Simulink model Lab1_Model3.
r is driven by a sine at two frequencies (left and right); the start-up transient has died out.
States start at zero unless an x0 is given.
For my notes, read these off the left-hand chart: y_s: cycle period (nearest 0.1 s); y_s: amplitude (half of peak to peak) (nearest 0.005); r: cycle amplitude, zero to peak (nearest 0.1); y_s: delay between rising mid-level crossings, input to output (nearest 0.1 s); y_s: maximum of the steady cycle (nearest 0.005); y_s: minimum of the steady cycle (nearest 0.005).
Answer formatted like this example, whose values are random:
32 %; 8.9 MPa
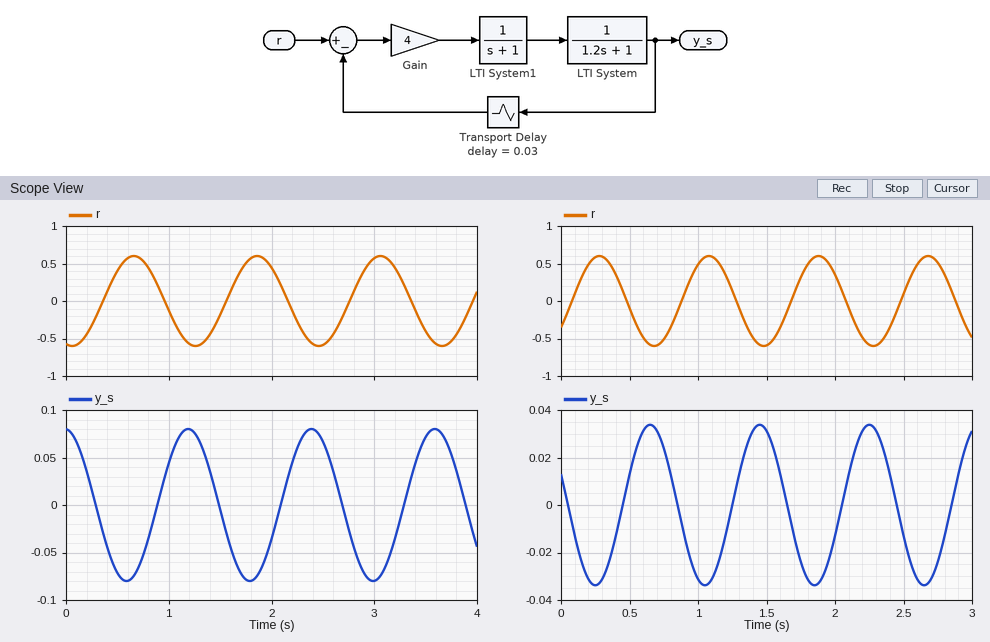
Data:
1.2 s; 0.080; 0.6; 0.5 s; 0.080; -0.080
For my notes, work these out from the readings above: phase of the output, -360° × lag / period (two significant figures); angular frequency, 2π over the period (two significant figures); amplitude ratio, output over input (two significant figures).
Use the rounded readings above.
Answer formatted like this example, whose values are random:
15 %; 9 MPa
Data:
-150°; 5.2 rad/s; 0.13
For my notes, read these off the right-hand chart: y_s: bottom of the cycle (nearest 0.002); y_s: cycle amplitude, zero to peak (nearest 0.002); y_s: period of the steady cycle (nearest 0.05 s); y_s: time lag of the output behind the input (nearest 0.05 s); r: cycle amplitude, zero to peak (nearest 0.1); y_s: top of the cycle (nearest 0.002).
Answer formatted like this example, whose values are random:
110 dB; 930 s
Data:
-0.034; 0.034; 0.80 s; 0.35 s; 0.6; 0.034
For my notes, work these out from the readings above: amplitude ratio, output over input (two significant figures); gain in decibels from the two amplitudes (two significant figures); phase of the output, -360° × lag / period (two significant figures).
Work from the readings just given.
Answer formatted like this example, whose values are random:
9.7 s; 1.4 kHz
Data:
0.057; -25 dB; -160°
